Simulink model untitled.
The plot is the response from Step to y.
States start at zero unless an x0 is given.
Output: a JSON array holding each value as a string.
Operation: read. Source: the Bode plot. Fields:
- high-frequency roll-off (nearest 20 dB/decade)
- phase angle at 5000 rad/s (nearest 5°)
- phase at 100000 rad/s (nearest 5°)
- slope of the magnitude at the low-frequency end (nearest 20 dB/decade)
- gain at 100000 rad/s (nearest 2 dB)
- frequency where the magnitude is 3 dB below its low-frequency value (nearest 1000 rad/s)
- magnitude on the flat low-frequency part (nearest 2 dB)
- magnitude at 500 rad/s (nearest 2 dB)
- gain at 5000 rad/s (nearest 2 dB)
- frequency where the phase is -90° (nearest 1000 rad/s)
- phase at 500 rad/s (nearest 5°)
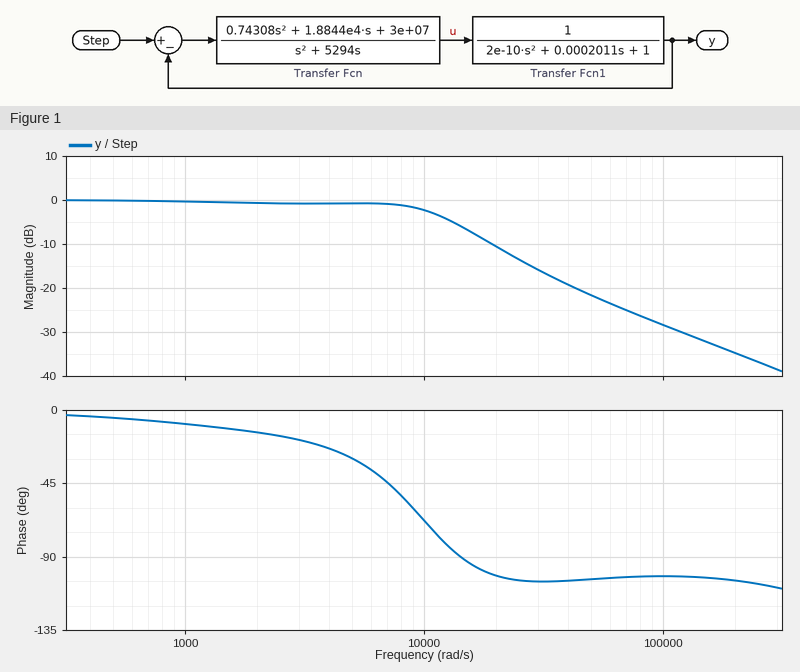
["-20 dB/decade", "-30°", "-100°", "0 dB/decade", "-28 dB", "11000 rad/s", "0 dB", "0 dB", "0 dB", "14000 rad/s", "-5°"]
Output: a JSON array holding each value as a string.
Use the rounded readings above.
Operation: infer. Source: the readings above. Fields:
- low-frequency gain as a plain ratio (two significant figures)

["1.0"]
